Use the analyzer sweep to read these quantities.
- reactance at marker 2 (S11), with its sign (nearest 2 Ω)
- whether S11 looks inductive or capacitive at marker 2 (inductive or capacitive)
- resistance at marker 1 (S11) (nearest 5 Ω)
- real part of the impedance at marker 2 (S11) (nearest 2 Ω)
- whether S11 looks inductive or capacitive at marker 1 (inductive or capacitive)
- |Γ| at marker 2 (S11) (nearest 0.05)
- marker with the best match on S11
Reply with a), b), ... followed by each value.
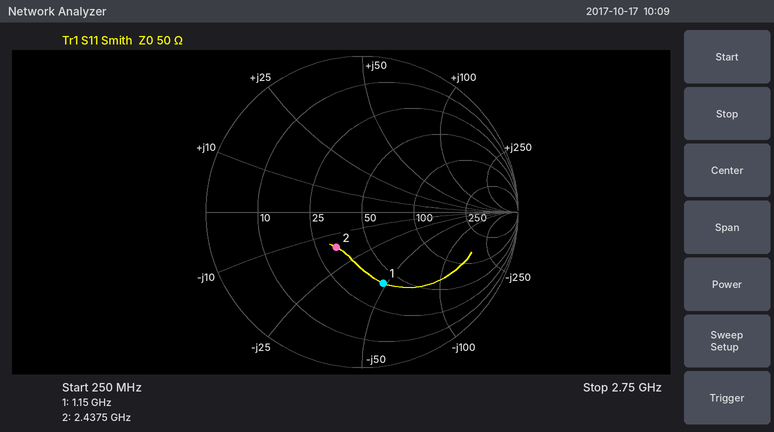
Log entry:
a) -16 Ω
b) capacitive
c) 40 Ω
d) 32 Ω
e) capacitive
f) 0.30
g) marker 2
